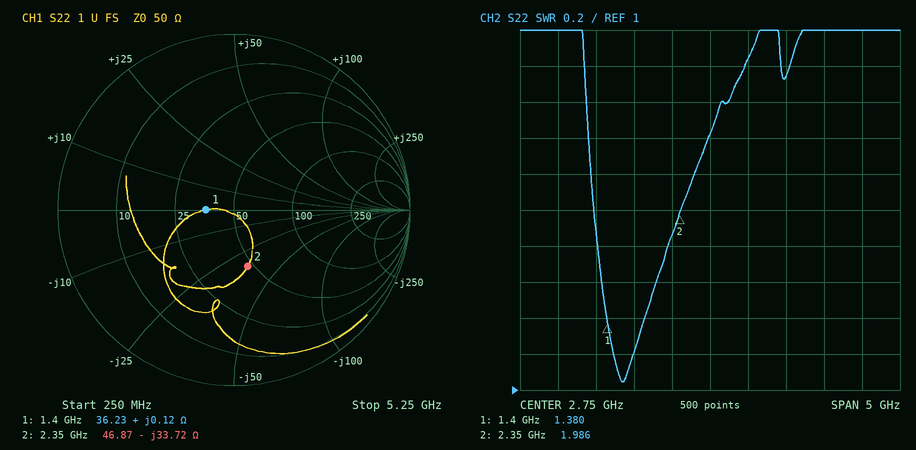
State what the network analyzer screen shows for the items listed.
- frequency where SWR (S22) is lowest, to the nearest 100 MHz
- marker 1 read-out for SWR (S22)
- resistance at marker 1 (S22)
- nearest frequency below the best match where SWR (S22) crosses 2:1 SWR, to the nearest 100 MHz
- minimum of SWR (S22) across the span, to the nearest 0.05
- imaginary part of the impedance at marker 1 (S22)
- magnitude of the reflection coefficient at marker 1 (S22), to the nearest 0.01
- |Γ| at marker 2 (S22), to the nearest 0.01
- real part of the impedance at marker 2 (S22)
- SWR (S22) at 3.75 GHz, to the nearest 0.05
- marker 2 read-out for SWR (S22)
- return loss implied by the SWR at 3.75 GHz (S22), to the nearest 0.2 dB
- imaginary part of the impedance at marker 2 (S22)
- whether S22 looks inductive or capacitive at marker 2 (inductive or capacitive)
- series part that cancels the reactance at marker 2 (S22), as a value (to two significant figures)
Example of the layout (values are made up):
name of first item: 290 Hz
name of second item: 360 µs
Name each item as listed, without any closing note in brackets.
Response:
frequency where SWR (S22) is lowest, to the nearest 100 MHz: 1.6 GHz
marker 1 read-out for SWR: 1.380
resistance at marker 1: 36.23 Ω
nearest frequency below the best match where SWR (S22) crosses 2:1 SWR, to the nearest 100 MHz: 1.2 GHz
minimum of SWR (S22) across the span, to the nearest 0.05: 1.05
imaginary part of the impedance at marker 1: +0.12 Ω
magnitude of the reflection coefficient at marker 1 (S22), to the nearest 0.01: 0.16
|Γ| at marker 2 (S22), to the nearest 0.01: 0.33
real part of the impedance at marker 2: 46.87 Ω
SWR (S22) at 3.75 GHz, to the nearest 0.05: 2.75
marker 2 read-out for SWR: 1.986
return loss implied by the SWR at 3.75 GHz (S22), to the nearest 0.2 dB: 6.6 dB
imaginary part of the impedance at marker 2: -33.72 Ω
whether S22 looks inductive or capacitive at marker 2: capacitive
series part that cancels the reactance at marker 2 (S22), as a value: 2.3 nH
